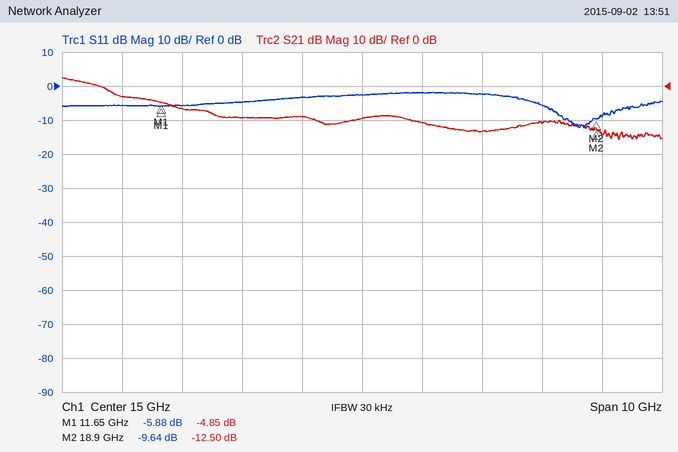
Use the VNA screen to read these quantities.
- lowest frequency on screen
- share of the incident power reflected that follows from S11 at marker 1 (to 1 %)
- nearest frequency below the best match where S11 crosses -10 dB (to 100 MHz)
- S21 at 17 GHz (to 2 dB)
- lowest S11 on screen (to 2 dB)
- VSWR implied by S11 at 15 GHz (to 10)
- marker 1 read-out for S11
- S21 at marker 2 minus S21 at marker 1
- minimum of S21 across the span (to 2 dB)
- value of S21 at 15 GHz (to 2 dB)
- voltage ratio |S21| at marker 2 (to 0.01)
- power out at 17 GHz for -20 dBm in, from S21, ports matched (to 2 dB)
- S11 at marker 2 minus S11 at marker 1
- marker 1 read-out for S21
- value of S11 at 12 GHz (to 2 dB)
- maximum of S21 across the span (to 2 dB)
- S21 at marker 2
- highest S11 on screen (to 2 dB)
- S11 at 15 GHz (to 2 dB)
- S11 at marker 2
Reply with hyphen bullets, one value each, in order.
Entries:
- 10 GHz
- 26 %
- 18.4 GHz
- -14 dB
- -12 dB
- 10
- -5.88 dB
- -7.65 dB
- -16 dB
- -10 dB
- 0.24
- -34 dBm
- -3.76 dB
- -4.85 dB
- -6 dB
- 2 dB
- -12.50 dB
- -2 dB
- -2 dB
- -9.64 dB
